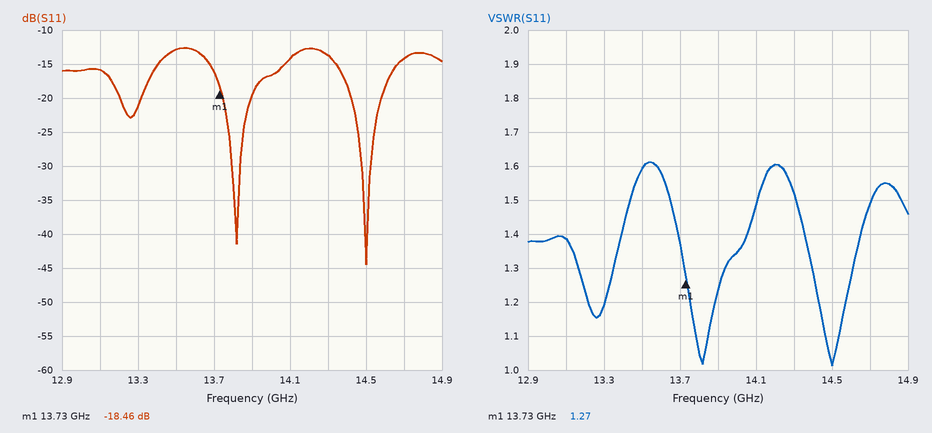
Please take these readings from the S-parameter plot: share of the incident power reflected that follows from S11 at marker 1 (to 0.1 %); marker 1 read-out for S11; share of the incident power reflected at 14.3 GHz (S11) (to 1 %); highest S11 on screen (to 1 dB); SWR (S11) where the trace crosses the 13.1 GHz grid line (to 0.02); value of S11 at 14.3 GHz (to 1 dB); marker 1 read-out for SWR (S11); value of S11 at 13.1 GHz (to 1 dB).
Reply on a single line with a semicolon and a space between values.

1.4 %; -18.46 dB; 4 %; -13 dB; 1.38; -14 dB; 1.27; -16 dB
